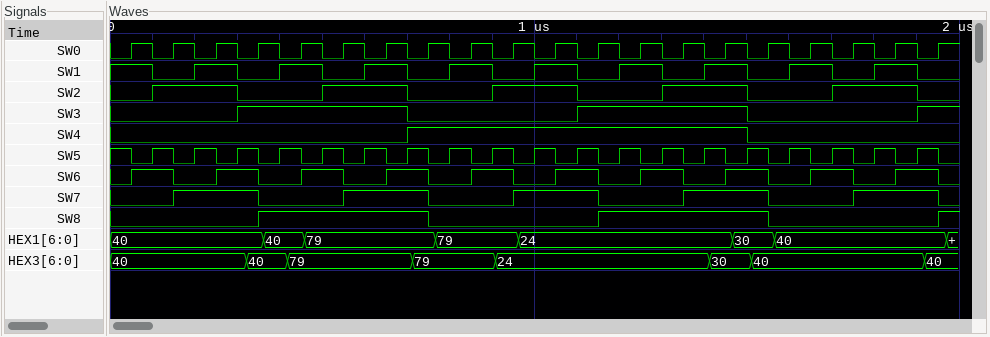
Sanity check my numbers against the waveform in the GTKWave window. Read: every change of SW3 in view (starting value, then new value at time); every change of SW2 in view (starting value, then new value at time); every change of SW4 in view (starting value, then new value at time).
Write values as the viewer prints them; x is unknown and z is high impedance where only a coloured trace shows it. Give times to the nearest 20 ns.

0, 1 at 300 ns, 0 at 700 ns, 1 at 1100 ns, 0 at 1500 ns, 1 at 1900 ns
0, 1 at 100 ns, 0 at 300 ns, 1 at 500 ns, 0 at 700 ns, 1 at 900 ns, 0 at 1100 ns, 1 at 1300 ns, 0 at 1500 ns, 1 at 1700 ns, 0 at 1900 ns
0, 1 at 700 ns, 0 at 1500 ns
